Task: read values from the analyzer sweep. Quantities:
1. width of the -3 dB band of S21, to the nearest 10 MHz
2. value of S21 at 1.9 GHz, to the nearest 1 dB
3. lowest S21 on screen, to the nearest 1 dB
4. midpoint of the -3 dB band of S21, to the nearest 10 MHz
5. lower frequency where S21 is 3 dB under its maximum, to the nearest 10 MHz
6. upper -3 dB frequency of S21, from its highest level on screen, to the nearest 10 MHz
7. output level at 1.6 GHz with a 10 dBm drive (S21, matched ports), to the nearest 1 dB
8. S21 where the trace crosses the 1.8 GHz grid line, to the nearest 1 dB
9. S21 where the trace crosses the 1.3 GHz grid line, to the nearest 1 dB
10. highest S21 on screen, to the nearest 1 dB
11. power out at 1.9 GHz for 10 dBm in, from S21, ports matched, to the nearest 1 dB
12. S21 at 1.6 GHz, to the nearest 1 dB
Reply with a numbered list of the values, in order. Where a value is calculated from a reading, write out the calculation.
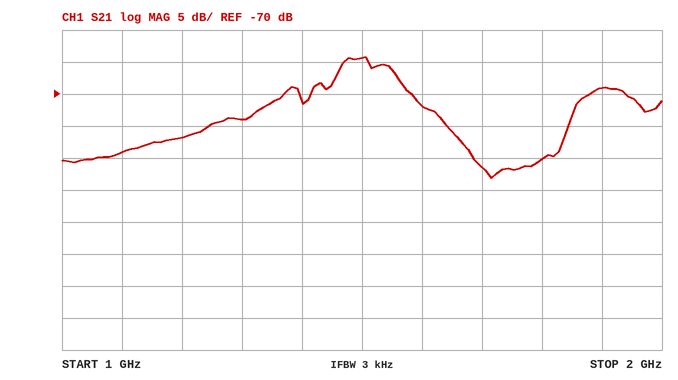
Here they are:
1. 1.56 GHz − 1.46 GHz = 100 MHz
2. -69 dB
3. -83 dB
4. 1.51 GHz
5. 1.46 GHz
6. 1.56 GHz
7. 10 dBm + (-72 dB) = -62 dBm
8. -80 dB
9. -74 dB
10. -64 dB
11. 10 dBm + (-69 dB) = -59 dBm
12. -72 dB
